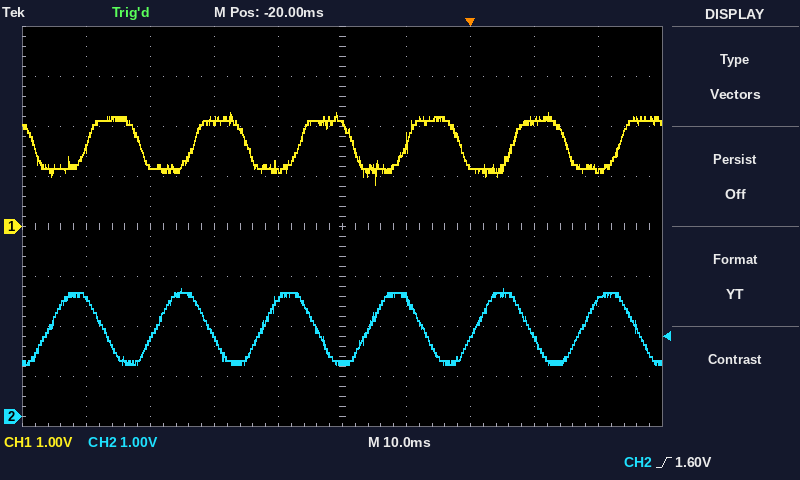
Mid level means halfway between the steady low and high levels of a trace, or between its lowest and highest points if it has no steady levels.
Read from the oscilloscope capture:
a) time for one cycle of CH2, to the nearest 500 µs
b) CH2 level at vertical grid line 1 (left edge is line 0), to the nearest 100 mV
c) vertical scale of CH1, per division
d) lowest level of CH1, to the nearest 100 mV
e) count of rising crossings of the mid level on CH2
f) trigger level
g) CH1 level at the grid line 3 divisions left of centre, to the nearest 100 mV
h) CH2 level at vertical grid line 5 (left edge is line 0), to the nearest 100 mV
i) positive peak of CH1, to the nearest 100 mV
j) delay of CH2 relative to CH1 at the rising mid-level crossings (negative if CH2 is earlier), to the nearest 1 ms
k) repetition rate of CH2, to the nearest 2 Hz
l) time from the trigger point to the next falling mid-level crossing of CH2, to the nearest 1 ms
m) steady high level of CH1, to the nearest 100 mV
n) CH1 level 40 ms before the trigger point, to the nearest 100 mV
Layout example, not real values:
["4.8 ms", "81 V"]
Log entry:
["16.5 ms", "2.4 V", "1 V", "800 mV", "6", "1.60 V", "1.2 V", "1.1 V", "2.3 V", "-6 ms", "60 Hz", "9 ms", "2.1 V", "2.1 V"]
